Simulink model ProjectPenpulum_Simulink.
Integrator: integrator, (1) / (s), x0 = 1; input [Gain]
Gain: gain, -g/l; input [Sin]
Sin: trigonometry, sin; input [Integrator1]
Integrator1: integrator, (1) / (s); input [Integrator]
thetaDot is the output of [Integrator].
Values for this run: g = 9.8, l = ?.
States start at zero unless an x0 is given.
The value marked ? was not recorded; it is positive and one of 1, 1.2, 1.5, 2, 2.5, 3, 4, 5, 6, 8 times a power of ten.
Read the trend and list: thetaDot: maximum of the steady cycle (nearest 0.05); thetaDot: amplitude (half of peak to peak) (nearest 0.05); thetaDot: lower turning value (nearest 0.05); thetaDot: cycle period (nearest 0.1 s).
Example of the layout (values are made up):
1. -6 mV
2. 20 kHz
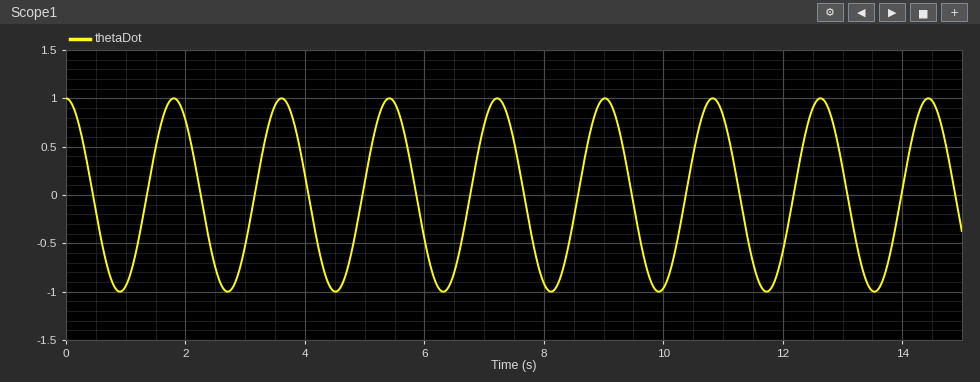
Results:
1. 1.00
2. 1.00
3. -1.00
4. 1.8 s
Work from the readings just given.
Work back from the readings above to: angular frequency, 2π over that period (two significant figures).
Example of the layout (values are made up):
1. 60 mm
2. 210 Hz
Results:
1. 3.5 rad/s
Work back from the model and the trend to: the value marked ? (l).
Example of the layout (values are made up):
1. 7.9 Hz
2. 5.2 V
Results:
1. 0.8
